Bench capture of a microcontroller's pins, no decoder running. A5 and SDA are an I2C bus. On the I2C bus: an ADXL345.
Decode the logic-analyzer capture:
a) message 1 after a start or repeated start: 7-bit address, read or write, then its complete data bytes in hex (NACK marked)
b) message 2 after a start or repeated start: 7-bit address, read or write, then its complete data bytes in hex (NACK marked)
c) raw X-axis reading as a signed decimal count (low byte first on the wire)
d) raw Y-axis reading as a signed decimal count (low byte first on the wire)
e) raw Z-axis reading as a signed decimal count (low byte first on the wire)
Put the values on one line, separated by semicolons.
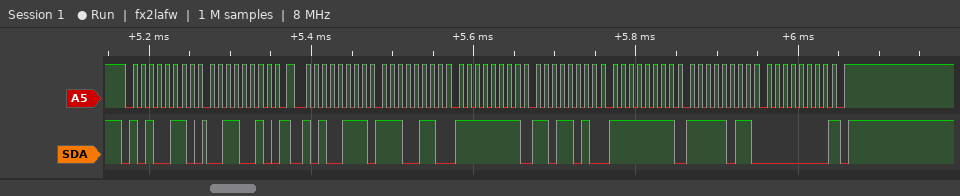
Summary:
0x53 write: 32; 0x53 read: E6 FF DA FF FB 00 NACK; -26; -38; 251
